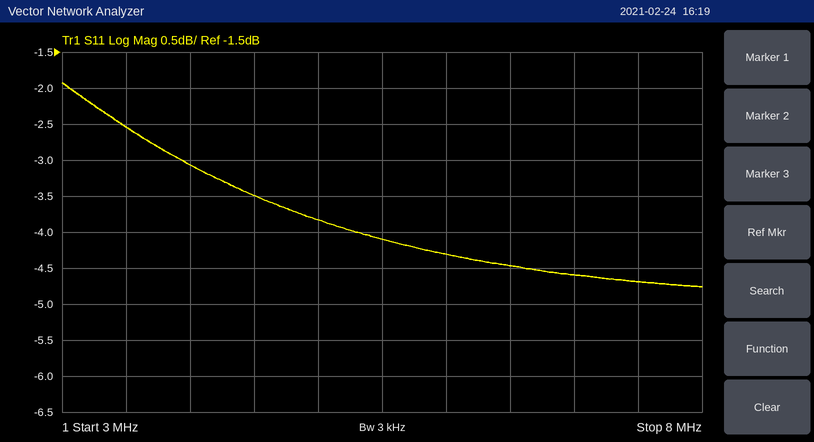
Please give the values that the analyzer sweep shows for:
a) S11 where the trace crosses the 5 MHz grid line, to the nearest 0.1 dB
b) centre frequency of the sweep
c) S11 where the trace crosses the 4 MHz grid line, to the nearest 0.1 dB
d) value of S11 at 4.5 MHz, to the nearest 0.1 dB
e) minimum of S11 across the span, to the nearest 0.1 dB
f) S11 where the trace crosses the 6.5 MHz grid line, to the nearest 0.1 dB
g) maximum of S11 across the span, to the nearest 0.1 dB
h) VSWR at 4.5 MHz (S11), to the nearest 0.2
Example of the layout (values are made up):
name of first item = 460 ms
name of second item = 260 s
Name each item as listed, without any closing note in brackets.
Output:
S11 where the trace crosses the 5 MHz grid line, to the nearest 0.1 dB = -3.8 dB
centre frequency of the sweep = 5.5 MHz
S11 where the trace crosses the 4 MHz grid line, to the nearest 0.1 dB = -3.1 dB
value of S11 at 4.5 MHz, to the nearest 0.1 dB = -3.5 dB
minimum of S11 across the span, to the nearest 0.1 dB = -4.8 dB
S11 where the trace crosses the 6.5 MHz grid line, to the nearest 0.1 dB = -4.5 dB
maximum of S11 across the span, to the nearest 0.1 dB = -1.9 dB
VSWR at 4.5 MHz (S11), to the nearest 0.2 = 5.0
